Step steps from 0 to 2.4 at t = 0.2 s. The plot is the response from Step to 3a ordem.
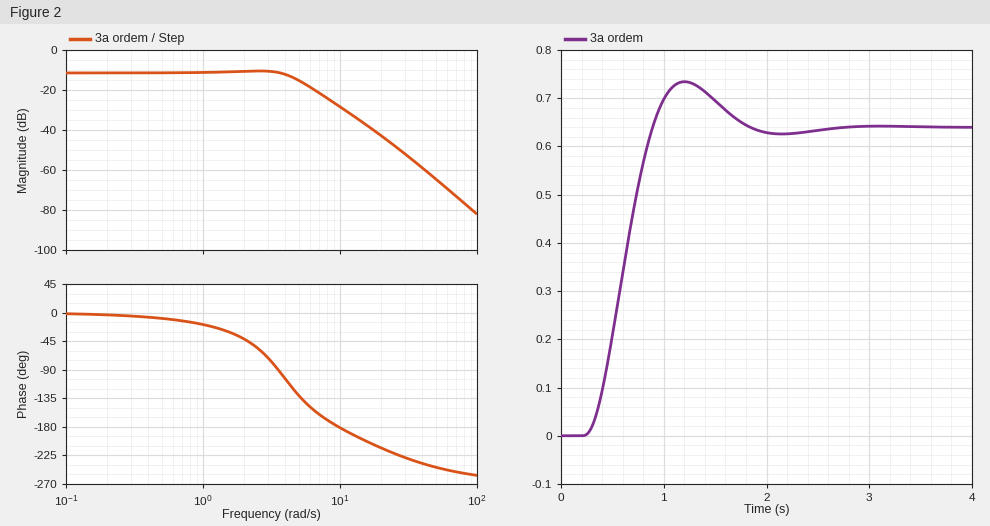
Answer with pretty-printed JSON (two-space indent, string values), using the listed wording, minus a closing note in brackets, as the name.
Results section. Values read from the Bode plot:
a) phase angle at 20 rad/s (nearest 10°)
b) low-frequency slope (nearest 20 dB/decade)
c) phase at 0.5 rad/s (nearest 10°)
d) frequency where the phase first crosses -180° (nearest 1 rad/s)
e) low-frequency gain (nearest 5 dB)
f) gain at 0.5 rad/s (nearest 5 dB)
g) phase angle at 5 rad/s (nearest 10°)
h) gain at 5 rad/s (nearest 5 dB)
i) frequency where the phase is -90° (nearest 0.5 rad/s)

{
  "phase angle at 20 rad/s": "-210°",
  "low-frequency slope": "0 dB/decade",
  "phase at 0.5 rad/s": "-10°",
  "frequency where the phase first crosses -180°": "10 rad/s",
  "low-frequency gain": "-10 dB",
  "gain at 0.5 rad/s": "-10 dB",
  "phase angle at 5 rad/s": "-130°",
  "gain at 5 rad/s": "-15 dB",
  "frequency where the phase is -90°": "3.5 rad/s"
}
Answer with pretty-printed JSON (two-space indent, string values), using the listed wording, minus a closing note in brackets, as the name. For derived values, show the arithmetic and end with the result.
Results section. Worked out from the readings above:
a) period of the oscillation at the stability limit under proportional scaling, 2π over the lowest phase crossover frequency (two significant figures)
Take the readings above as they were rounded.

{
  "period of the oscillation at the stability limit under proportional scaling, 2π over the lowest phase crossover frequency": "2π / 10 = 0.63 s"
}
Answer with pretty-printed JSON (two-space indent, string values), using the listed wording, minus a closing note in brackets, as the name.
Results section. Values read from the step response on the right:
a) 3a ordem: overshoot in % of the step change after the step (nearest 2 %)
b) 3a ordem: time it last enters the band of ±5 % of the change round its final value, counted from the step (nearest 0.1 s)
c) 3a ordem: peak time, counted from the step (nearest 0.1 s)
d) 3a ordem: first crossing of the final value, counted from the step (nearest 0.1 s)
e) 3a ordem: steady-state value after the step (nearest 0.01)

{
  "3a ordem: overshoot in % of the step change after the step": "14 %",
  "3a ordem: time it last enters the band of ±5 % of the change round its final value, counted from the step": "1.4 s",
  "3a ordem: peak time, counted from the step": "1.0 s",
  "3a ordem: first crossing of the final value, counted from the step": "0.7 s",
  "3a ordem: steady-state value after the step": "0.64"
}
